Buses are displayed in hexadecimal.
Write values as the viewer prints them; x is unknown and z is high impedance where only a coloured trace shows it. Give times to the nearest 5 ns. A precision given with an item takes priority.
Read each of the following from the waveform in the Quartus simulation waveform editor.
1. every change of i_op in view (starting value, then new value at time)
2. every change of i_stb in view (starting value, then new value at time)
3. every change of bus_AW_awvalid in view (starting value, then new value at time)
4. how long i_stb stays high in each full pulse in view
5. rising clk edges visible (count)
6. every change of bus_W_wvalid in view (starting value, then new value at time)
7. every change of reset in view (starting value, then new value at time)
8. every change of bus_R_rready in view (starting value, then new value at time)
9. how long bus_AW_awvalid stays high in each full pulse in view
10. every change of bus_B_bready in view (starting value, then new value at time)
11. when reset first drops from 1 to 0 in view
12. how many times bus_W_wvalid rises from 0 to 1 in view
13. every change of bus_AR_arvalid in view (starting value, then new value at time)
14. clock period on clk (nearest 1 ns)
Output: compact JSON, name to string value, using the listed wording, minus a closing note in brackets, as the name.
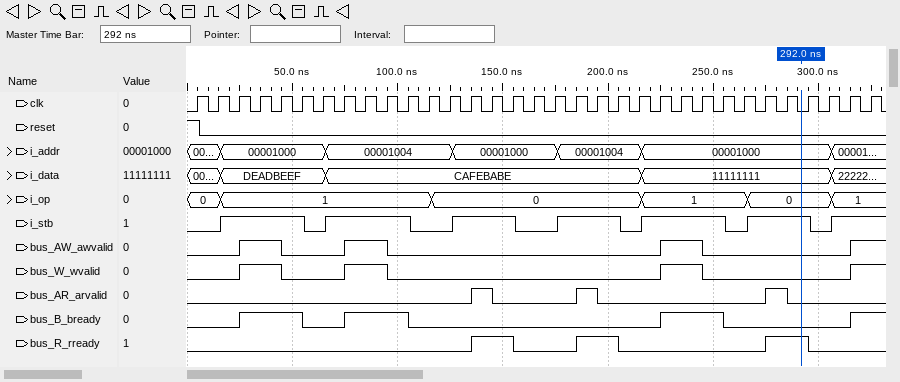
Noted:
{"every change of i_op in view": "0, 1 at 15 ns, 0 at 115 ns, 1 at 215 ns, 0 at 265 ns, 1 at 305 ns", "every change of i_stb in view": "0, 1 at 15 ns, 0 at 55 ns, 1 at 65 ns, 0 at 105 ns, 1 at 125 ns, 0 at 155 ns, 1 at 175 ns, 0 at 205 ns, 1 at 215 ns, 0 at 255 ns, 1 at 265 ns, 0 at 295 ns, 1 at 305 ns", "every change of bus_AW_awvalid in view": "0, 1 at 25 ns, 0 at 45 ns, 1 at 75 ns, 0 at 95 ns, 1 at 225 ns, 0 at 245 ns, 1 at 315 ns", "how long i_stb stays high in each full pulse in view": "40 ns, 40 ns, 30 ns, 30 ns, 40 ns, 30 ns", "rising clk edges visible": "33", "every change of bus_W_wvalid in view": "0, 1 at 25 ns, 0 at 45 ns, 1 at 75 ns, 0 at 95 ns, 1 at 225 ns, 0 at 245 ns, 1 at 315 ns", "every change of reset in view": "1, 0 at 5 ns", "every change of bus_R_rready in view": "0, 1 at 135 ns, 0 at 155 ns, 1 at 185 ns, 0 at 205 ns, 1 at 275 ns, 0 at 295 ns", "how long bus_AW_awvalid stays high in each full pulse in view": "20 ns, 20 ns, 20 ns", "every change of bus_B_bready in view": "0, 1 at 25 ns, 0 at 55 ns, 1 at 75 ns, 0 at 105 ns, 1 at 225 ns, 0 at 255 ns, 1 at 315 ns", "when reset first drops from 1 to 0 in view": "5 ns", "how many times bus_W_wvalid rises from 0 to 1 in view": "4", "every change of bus_AR_arvalid in view": "0, 1 at 135 ns, 0 at 145 ns, 1 at 185 ns, 0 at 195 ns, 1 at 275 ns, 0 at 285 ns", "clock period on clk": "10 ns"}
